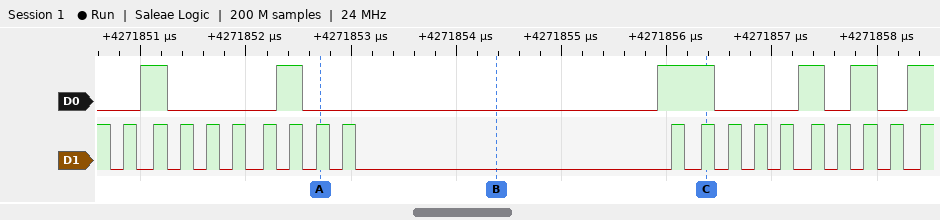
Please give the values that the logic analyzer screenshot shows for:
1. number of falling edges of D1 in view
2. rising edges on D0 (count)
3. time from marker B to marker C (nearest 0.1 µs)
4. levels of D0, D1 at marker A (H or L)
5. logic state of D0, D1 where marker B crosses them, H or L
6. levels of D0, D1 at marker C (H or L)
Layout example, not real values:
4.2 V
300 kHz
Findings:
19
6
2 µs
D0=L, D1=H
D0=L, D1=L
D0=H, D1=H
